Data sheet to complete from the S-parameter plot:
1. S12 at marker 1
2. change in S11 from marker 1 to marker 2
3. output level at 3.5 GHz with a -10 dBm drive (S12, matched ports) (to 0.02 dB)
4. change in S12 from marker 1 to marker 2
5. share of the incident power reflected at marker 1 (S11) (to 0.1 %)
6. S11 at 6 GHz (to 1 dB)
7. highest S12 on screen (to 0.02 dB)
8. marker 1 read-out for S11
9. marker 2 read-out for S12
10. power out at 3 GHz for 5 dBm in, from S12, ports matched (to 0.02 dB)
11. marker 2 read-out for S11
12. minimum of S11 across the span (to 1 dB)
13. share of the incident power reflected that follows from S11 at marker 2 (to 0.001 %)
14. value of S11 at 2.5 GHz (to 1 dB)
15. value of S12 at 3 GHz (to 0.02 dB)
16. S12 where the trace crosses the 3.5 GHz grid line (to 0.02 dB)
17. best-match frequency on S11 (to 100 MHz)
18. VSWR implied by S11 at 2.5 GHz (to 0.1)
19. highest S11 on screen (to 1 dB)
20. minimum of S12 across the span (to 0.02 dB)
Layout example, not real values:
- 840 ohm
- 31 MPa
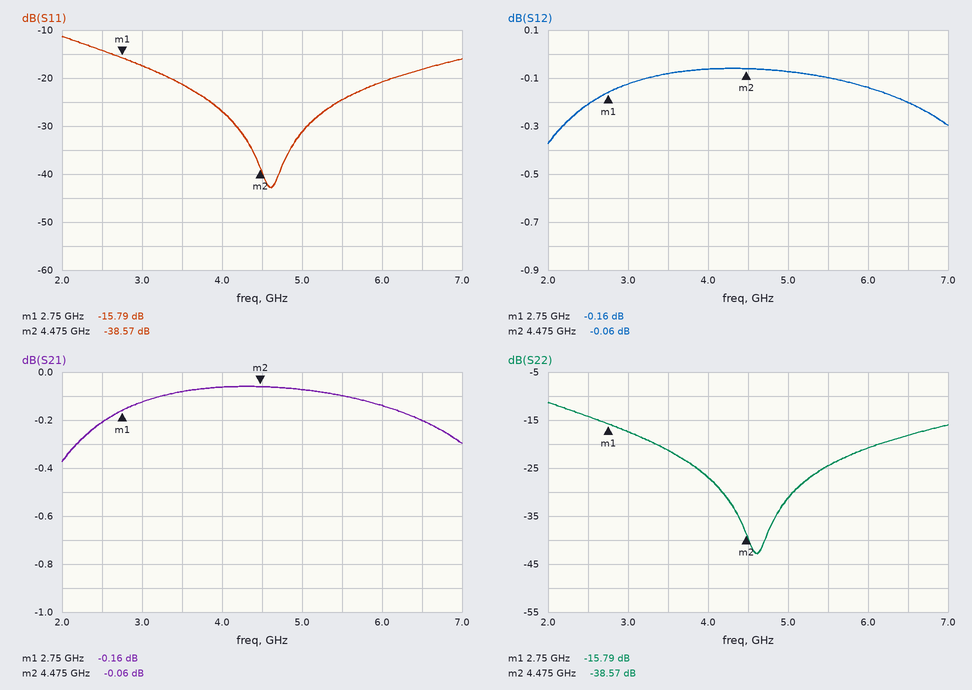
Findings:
- -0.16 dB
- -22.78 dB
- -10.08 dBm
- 0.10 dB
- 2.6 %
- -21 dB
- -0.06 dB
- -15.79 dB
- -0.06 dB
- 4.88 dBm
- -38.57 dB
- -43 dB
- 0.014 %
- -14 dB
- -0.12 dB
- -0.08 dB
- 4.6 GHz
- 1.5
- -11 dB
- -0.38 dB
